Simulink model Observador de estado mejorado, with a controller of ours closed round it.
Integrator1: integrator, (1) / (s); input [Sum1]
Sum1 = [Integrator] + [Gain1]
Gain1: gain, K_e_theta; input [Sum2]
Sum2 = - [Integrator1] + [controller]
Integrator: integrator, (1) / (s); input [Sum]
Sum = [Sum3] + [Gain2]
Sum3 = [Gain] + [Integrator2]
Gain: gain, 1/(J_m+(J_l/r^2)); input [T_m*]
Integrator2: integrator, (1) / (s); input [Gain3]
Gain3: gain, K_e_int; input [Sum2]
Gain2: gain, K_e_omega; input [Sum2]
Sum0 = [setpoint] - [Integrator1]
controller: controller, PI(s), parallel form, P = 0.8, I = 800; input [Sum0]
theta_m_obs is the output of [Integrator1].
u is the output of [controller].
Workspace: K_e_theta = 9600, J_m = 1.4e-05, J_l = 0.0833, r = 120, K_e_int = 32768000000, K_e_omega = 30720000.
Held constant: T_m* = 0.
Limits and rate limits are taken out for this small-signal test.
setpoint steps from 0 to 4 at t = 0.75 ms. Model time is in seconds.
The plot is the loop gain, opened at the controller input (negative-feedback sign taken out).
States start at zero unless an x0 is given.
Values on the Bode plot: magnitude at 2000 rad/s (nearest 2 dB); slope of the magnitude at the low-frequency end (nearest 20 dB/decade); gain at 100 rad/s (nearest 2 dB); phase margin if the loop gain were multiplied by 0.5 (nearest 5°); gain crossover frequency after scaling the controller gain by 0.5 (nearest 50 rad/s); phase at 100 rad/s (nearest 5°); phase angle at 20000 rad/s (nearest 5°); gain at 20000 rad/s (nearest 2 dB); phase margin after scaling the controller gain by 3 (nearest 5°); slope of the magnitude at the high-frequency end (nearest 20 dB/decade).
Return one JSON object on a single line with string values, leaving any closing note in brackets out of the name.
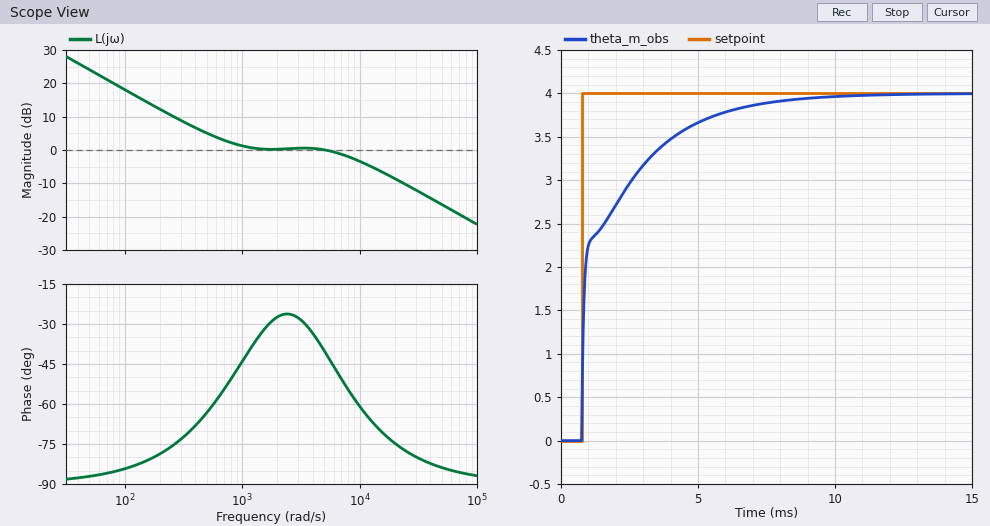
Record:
{"magnitude at 2000 rad/s": "0 dB", "slope of the magnitude at the low-frequency end": "-20 dB/decade", "gain at 100 rad/s": "18 dB", "phase margin if the loop gain were multiplied by 0.5": "115°", "gain crossover frequency after scaling the controller gain by 0.5": "450 rad/s", "phase at 100 rad/s": "-85°", "phase angle at 20000 rad/s": "-75°", "gain at 20000 rad/s": "-8 dB", "phase margin after scaling the controller gain by 3": "105°", "slope of the magnitude at the high-frequency end": "-20 dB/decade"}
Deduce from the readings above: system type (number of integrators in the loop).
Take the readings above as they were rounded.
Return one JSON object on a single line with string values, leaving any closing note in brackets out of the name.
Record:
{"system type": "1"}
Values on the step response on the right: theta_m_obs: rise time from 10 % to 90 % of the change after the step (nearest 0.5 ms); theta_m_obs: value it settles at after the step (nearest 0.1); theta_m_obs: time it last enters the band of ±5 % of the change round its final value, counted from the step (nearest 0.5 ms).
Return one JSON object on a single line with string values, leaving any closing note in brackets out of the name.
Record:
{"theta_m_obs: rise time from 10 % to 90 % of the change after the step": "4.0 ms", "theta_m_obs: value it settles at after the step": "4.0", "theta_m_obs: time it last enters the band of ±5 % of the change round its final value, counted from the step": "5.5 ms"}
